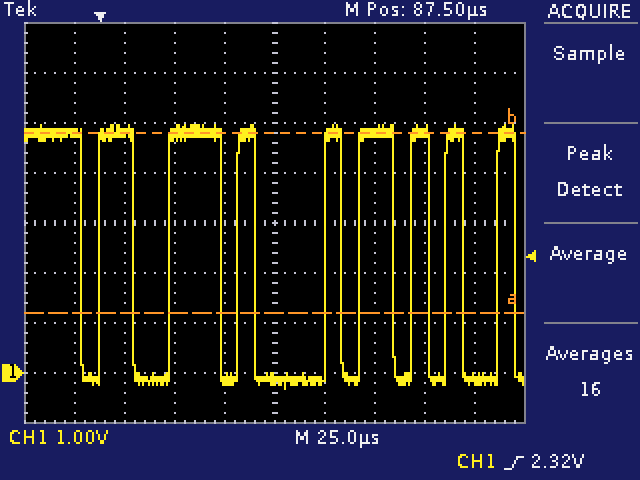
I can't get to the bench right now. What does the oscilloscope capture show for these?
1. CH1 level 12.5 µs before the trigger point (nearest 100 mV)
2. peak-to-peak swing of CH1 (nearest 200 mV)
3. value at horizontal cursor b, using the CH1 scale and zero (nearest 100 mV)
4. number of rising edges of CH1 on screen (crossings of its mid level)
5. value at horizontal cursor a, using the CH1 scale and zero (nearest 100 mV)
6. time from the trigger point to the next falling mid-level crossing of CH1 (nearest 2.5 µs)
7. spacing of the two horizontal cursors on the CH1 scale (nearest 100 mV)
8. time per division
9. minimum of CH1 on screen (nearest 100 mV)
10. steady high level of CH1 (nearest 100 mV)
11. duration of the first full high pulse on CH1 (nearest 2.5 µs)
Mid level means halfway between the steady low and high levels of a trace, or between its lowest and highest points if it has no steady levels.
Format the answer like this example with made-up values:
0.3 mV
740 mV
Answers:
4.8 V
5.2 V
4.8 V
8
1.2 V
17.5 µs
3.6 V
25 µs
-300 mV
4.8 V
17.5 µs
